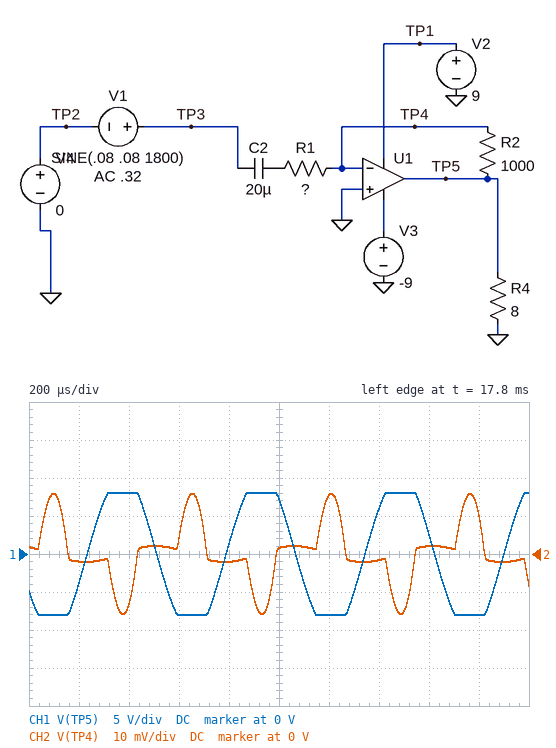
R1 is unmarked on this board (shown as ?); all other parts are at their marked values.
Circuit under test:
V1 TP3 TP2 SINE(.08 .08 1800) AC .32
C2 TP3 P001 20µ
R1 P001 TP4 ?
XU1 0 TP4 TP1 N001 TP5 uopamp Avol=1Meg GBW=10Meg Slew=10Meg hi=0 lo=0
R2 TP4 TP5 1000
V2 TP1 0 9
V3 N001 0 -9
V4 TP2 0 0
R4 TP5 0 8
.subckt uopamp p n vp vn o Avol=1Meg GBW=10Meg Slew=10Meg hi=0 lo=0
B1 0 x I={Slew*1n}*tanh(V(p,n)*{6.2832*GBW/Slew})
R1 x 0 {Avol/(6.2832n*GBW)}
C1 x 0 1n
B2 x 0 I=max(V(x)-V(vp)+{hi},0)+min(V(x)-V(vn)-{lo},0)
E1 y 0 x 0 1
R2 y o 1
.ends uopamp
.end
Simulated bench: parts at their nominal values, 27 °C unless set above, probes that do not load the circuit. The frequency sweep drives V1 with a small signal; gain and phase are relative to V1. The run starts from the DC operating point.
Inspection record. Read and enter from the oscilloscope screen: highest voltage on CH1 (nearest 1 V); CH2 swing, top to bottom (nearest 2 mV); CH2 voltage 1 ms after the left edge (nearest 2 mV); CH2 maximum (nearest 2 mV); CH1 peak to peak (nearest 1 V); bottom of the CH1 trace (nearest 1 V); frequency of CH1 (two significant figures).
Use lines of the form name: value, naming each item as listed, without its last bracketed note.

highest voltage on CH1: 8 V
CH2 swing, top to bottom: 32 mV
CH2 voltage 1 ms after the left edge: 2 mV
CH2 maximum: 16 mV
CH1 peak to peak: 16 V
bottom of the CH1 trace: -8 V
frequency of CH1: 1.8 kHz
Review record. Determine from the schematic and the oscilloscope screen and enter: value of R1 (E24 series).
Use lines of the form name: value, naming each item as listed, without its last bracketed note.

value of R1: 6.8 Ω
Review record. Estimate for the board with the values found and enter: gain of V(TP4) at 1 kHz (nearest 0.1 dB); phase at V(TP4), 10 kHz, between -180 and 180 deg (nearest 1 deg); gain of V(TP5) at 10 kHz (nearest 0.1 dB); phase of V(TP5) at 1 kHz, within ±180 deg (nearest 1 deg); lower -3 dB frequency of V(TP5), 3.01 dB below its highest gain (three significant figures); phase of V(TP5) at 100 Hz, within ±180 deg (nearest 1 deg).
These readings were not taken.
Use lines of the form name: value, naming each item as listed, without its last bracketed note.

gain of V(TP4) at 1 kHz: -39.3 dB
phase at V(TP4), 10 kHz, between -180 and 180 deg: 87 deg
gain of V(TP5) at 10 kHz: 43.3 dB
phase of V(TP5) at 1 kHz, within ±180 deg: -131 deg
lower -3 dB frequency of V(TP5), 3.01 dB below its highest gain: 1.15 kHz
phase of V(TP5) at 100 Hz, within ±180 deg: -95 deg
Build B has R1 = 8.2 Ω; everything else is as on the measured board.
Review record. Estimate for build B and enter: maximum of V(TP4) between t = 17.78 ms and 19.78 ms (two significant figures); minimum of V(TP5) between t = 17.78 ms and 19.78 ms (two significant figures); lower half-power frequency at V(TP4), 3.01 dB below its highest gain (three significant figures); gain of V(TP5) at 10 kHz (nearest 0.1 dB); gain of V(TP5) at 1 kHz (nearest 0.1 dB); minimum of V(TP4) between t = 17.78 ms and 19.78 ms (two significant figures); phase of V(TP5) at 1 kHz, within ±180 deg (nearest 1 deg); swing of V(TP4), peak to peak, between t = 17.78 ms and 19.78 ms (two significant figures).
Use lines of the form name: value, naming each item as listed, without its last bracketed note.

maximum of V(TP4) between t = 17.78 ms and 19.78 ms: 6.0 mV
minimum of V(TP5) between t = 17.78 ms and 19.78 ms: -8.0 V
lower half-power frequency at V(TP4), 3.01 dB below its highest gain: 71.3 kHz
gain of V(TP5) at 10 kHz: 41.7 dB
gain of V(TP5) at 1 kHz: 38.9 dB
minimum of V(TP4) between t = 17.78 ms and 19.78 ms: -6.0 mV
phase of V(TP5) at 1 kHz, within ±180 deg: -136 deg
swing of V(TP4), peak to peak, between t = 17.78 ms and 19.78 ms: 12 mV
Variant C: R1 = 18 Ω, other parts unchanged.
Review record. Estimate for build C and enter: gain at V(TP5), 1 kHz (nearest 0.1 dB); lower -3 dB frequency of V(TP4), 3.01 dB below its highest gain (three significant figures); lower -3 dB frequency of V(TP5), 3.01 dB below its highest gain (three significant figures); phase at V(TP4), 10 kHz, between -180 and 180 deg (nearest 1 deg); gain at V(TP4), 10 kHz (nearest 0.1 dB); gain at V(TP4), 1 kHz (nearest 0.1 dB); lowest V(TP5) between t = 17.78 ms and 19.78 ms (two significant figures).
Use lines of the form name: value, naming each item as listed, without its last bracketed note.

gain at V(TP5), 1 kHz: 34.1 dB
lower -3 dB frequency of V(TP4), 3.01 dB below its highest gain: 157 kHz
lower -3 dB frequency of V(TP5), 3.01 dB below its highest gain: 441 Hz
phase at V(TP4), 10 kHz, between -180 and 180 deg: 89 deg
gain at V(TP4), 10 kHz: -24.1 dB
gain at V(TP4), 1 kHz: -44.8 dB
lowest V(TP5) between t = 17.78 ms and 19.78 ms: -4.3 V
